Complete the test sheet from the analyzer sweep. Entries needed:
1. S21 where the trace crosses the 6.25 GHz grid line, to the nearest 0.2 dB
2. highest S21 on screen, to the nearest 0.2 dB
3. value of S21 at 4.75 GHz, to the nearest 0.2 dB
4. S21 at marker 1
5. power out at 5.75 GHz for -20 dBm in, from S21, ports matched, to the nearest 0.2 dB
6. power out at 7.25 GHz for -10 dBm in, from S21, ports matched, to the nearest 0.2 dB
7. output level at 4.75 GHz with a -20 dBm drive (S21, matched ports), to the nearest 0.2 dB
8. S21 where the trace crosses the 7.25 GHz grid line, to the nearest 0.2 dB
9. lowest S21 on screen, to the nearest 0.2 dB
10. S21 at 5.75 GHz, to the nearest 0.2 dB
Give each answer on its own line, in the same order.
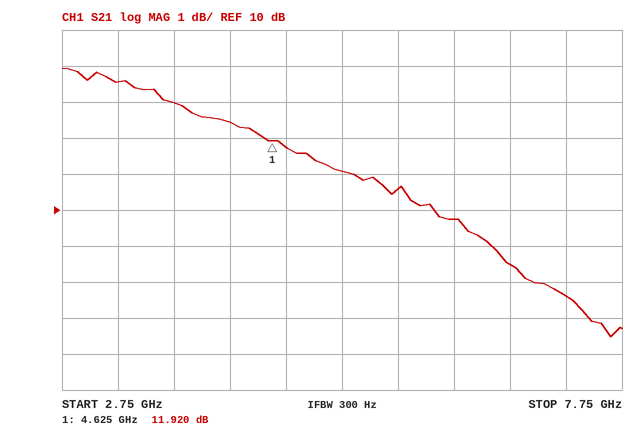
9.8 dB
14.0 dB
11.8 dB
11.920 dB
-9.4 dBm
-2.4 dBm
-8.2 dBm
7.6 dB
6.4 dB
10.6 dB
